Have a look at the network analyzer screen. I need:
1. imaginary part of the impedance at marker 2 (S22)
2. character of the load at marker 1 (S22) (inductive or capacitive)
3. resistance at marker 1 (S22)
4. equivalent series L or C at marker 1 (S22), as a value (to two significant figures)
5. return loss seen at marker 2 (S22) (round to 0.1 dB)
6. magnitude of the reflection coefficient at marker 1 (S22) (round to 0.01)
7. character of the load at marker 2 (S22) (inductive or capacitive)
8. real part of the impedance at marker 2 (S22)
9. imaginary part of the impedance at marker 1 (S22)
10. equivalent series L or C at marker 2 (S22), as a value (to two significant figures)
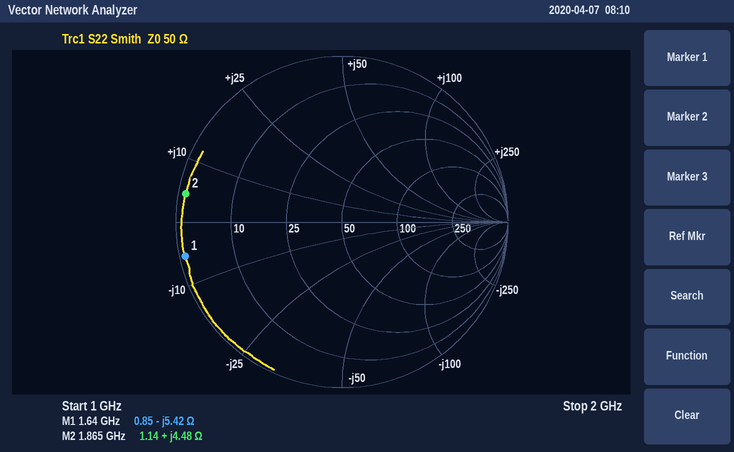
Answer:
+4.48 Ω
capacitive
0.85 Ω
18 pF
0.4 dB
0.97
inductive
1.14 Ω
-5.42 Ω
380 pH
